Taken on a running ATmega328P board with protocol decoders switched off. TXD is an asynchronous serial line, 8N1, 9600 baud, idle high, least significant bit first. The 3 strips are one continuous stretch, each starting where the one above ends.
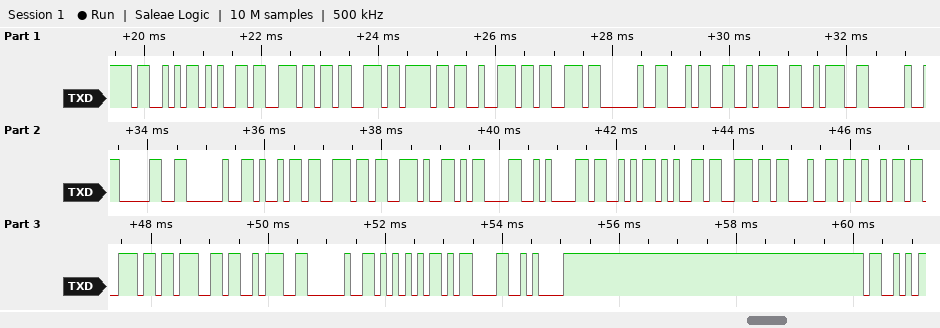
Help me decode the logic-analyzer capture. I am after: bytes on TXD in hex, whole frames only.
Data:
53 65 6E 73 6F 72 73 20 34 3A 3A 20 30 20 69 6E 2E 0D 0A 53 65 6E 64 69 6E 67 3A 20 55 0D 0A 53
